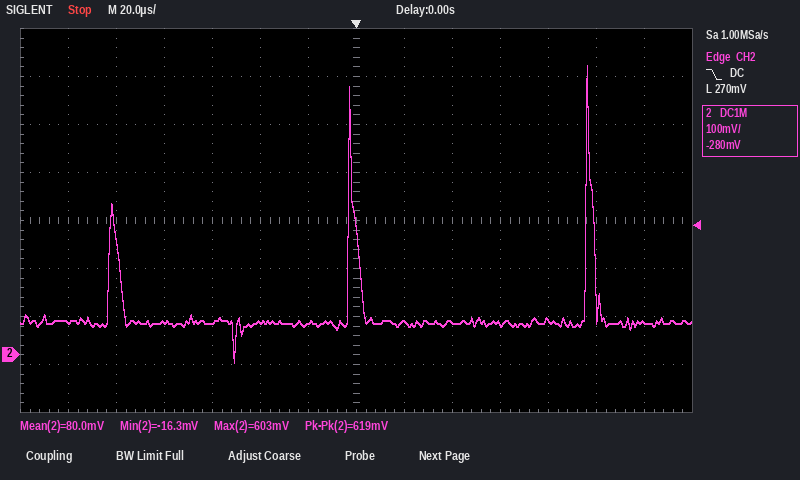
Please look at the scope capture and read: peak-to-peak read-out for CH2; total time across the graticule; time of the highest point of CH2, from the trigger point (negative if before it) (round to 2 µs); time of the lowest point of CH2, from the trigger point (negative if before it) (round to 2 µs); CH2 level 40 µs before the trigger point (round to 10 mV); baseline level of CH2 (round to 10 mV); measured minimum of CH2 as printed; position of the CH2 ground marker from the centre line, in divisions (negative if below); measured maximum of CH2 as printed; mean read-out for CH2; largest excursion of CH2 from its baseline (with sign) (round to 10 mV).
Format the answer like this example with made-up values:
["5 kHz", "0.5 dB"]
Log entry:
["619 mV", "280 µs", "+96 µs", "-50 µs", "70 mV", "70 mV", "-16.3 mV", "-2.8 div", "603 mV", "80.0 mV", "+540 mV"]
